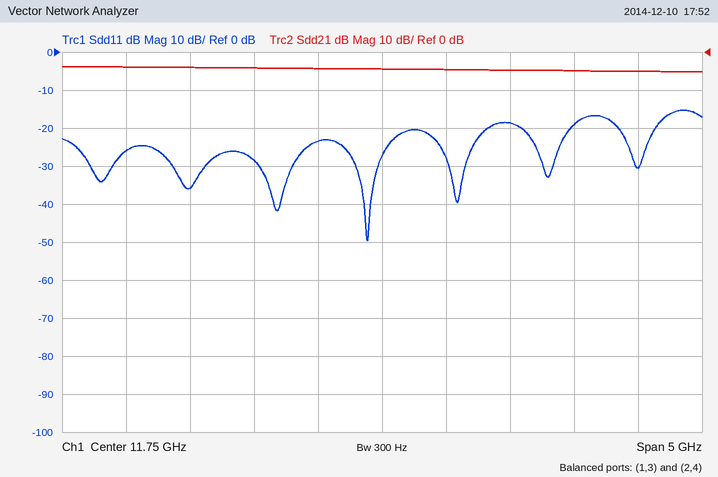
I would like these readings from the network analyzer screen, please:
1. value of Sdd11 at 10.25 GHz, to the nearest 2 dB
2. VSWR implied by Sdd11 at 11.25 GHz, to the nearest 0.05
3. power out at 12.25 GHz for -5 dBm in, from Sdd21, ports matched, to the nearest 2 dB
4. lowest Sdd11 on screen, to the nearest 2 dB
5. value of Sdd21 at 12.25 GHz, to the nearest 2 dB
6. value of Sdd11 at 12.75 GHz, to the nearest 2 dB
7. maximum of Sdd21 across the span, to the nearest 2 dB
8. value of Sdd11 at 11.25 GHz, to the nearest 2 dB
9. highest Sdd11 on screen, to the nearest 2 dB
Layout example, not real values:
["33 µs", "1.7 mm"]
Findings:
["-36 dB", "1.15", "-10 dBm", "-50 dB", "-4 dB", "-18 dB", "-4 dB", "-24 dB", "-16 dB"]
